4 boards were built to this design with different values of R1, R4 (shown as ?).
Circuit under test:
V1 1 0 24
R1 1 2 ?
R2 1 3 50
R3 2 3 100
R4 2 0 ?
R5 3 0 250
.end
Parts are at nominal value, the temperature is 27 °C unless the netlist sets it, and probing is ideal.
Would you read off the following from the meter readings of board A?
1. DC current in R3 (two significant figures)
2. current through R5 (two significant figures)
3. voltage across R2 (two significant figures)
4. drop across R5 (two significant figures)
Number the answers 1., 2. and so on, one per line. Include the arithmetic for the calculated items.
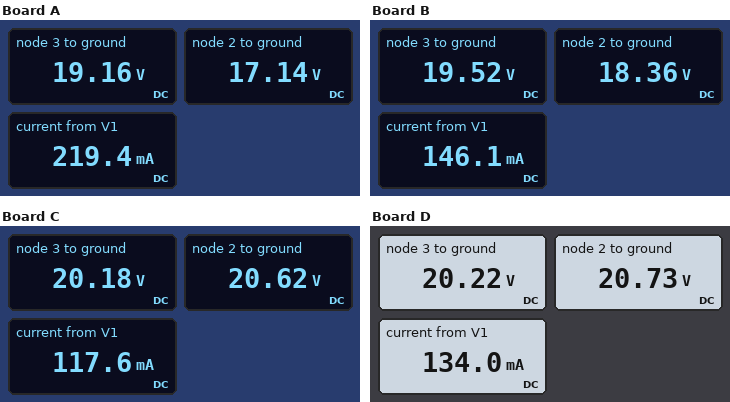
1. (19.16 V - 17.14 V) / 100 Ω = 20 mA
2. (19.16 V) / 250 Ω = 77 mA
3. 24 V - 19.16 V = 4.8 V
4. 19.16 V = 19 V
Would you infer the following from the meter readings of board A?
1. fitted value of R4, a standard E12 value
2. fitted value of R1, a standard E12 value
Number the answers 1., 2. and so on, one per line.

1. 120 Ω
2. 56 Ω
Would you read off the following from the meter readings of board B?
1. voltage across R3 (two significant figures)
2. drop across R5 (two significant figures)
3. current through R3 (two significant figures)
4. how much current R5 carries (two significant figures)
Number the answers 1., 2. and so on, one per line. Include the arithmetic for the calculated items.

1. 19.52 V - 18.36 V = 1.2 V
2. 19.52 V = 20 V
3. (19.52 V - 18.36 V) / 100 Ω = 12 mA
4. (19.52 V) / 250 Ω = 78 mA
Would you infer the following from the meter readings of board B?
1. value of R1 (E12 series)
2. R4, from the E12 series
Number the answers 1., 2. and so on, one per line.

1. 100 Ω
2. 270 Ω
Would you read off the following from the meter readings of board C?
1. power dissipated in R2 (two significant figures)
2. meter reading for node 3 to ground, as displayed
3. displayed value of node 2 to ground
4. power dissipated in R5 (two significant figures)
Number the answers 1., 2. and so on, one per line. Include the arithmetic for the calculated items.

1. (24 V - 20.18 V)^2 / 50 Ω = 290 mW
2. 20.18 V
3. 20.62 V
4. (20.18 V)^2 / 250 Ω = 1.6 W
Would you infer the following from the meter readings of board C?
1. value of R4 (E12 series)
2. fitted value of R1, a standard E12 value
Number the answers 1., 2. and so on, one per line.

1. 560 Ω
2. 82 Ω
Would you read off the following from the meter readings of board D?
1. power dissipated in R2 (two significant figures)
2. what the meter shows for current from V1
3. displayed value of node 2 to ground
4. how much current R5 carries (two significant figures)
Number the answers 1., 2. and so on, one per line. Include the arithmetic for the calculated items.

1. (24 V - 20.22 V)^2 / 50 Ω = 290 mW
2. 134.0 mA
3. 20.73 V
4. (20.22 V) / 250 Ω = 81 mA
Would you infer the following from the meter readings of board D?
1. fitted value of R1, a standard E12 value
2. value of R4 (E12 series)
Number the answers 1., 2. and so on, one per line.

1. 56 Ω
2. 390 Ω
